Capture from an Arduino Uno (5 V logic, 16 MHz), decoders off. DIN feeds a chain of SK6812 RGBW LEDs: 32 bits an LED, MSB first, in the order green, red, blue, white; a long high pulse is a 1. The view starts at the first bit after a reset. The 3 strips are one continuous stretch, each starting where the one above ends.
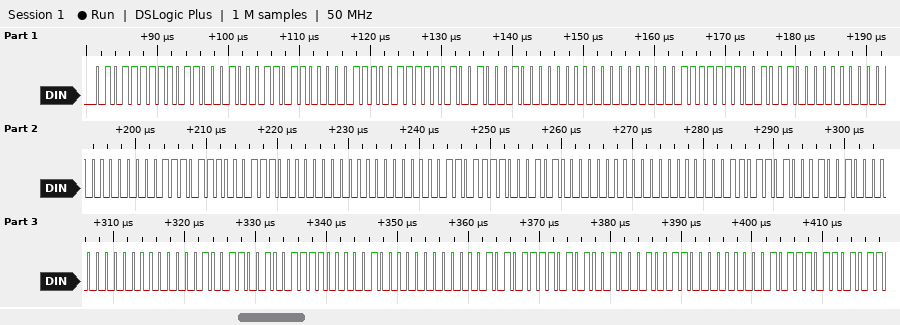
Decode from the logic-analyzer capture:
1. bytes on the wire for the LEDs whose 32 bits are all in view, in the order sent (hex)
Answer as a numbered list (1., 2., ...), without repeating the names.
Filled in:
1. 5F B1 1B 07 3E 91 00 00 3F 92 00 00 3B 8E 00 00 37 8A 00 00 36 89 00 00 4C 9E 08 00 57 A9 13 00
